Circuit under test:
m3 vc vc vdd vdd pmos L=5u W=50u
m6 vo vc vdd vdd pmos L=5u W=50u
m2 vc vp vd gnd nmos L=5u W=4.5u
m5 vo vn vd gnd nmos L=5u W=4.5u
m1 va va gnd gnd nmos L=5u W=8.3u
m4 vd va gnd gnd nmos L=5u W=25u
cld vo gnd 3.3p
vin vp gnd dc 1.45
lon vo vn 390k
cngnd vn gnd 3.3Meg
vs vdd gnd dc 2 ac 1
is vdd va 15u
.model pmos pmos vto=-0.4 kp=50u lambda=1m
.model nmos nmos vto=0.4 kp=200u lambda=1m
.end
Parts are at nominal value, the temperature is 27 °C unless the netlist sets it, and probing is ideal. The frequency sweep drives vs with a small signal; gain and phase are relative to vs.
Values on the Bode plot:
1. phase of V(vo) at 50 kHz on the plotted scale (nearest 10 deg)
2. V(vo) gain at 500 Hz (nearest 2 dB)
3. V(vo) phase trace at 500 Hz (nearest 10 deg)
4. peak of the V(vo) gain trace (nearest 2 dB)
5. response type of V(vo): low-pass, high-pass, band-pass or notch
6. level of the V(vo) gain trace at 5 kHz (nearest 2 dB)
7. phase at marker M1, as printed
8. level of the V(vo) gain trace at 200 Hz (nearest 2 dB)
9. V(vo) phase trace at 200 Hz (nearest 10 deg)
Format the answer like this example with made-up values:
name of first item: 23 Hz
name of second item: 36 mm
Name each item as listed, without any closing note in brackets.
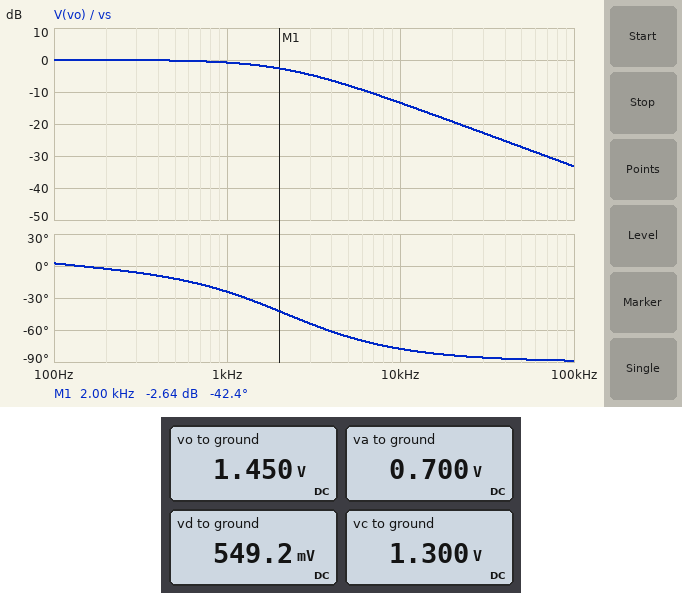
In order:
phase of V(vo) at 50 kHz on the plotted scale: -90 deg
V(vo) gain at 500 Hz: 0 dB
V(vo) phase trace at 500 Hz: -10 deg
peak of the V(vo) gain trace: 0 dB
response type of V(vo): low-pass, high-pass, band-pass or notch: low-pass
level of the V(vo) gain trace at 5 kHz: -8 dB
phase at marker M1, as printed: -42.4 deg
level of the V(vo) gain trace at 200 Hz: 0 dB
V(vo) phase trace at 200 Hz: 0 deg
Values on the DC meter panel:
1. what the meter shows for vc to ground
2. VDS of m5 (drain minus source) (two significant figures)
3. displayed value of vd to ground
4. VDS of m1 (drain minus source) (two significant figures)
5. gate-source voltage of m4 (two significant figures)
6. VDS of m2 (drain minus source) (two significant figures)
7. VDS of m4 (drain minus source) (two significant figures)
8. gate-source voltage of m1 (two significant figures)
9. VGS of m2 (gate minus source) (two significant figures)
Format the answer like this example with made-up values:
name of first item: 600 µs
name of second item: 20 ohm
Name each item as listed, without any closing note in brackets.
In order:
what the meter shows for vc to ground: 1.300 V
VDS of m5 (drain minus source): 900 mV
displayed value of vd to ground: 549.2 mV
VDS of m1 (drain minus source): 700 mV
gate-source voltage of m4: 700 mV
VDS of m2 (drain minus source): 750 mV
VDS of m4 (drain minus source): 550 mV
gate-source voltage of m1: 700 mV
VGS of m2 (gate minus source): 900 mV
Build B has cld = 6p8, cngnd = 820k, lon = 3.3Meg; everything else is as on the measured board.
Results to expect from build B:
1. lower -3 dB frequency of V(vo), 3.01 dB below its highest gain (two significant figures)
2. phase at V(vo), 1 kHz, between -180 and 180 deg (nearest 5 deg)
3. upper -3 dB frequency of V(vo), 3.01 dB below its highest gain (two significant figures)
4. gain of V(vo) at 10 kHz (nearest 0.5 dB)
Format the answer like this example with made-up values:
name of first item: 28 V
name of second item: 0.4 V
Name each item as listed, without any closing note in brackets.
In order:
lower -3 dB frequency of V(vo), 3.01 dB below its highest gain: 1.1 Hz
phase at V(vo), 1 kHz, between -180 and 180 deg: -45 deg
upper -3 dB frequency of V(vo), 3.01 dB below its highest gain: 1.1 kHz
gain of V(vo) at 10 kHz: -19.5 dB
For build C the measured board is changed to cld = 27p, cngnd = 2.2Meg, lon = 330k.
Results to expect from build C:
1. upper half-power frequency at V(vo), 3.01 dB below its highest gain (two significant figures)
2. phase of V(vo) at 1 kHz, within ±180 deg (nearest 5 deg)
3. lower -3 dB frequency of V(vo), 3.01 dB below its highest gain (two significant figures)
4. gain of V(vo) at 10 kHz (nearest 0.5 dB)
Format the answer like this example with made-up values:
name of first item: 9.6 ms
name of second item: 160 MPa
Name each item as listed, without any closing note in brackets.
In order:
upper half-power frequency at V(vo), 3.01 dB below its highest gain: 280 Hz
phase of V(vo) at 1 kHz, within ±180 deg: -75 deg
lower -3 dB frequency of V(vo), 3.01 dB below its highest gain: 10 Hz
gain of V(vo) at 10 kHz: -31.5 dB
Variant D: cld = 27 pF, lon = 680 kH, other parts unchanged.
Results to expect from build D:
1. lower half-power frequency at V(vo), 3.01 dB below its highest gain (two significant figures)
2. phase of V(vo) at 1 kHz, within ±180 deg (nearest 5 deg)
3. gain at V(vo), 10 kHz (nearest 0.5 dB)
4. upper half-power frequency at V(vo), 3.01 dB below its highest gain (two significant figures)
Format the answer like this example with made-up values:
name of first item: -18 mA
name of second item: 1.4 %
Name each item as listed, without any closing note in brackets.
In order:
lower half-power frequency at V(vo), 3.01 dB below its highest gain: 5.1 Hz
phase of V(vo) at 1 kHz, within ±180 deg: -75 deg
gain at V(vo), 10 kHz: -31.5 dB
upper half-power frequency at V(vo), 3.01 dB below its highest gain: 270 Hz
